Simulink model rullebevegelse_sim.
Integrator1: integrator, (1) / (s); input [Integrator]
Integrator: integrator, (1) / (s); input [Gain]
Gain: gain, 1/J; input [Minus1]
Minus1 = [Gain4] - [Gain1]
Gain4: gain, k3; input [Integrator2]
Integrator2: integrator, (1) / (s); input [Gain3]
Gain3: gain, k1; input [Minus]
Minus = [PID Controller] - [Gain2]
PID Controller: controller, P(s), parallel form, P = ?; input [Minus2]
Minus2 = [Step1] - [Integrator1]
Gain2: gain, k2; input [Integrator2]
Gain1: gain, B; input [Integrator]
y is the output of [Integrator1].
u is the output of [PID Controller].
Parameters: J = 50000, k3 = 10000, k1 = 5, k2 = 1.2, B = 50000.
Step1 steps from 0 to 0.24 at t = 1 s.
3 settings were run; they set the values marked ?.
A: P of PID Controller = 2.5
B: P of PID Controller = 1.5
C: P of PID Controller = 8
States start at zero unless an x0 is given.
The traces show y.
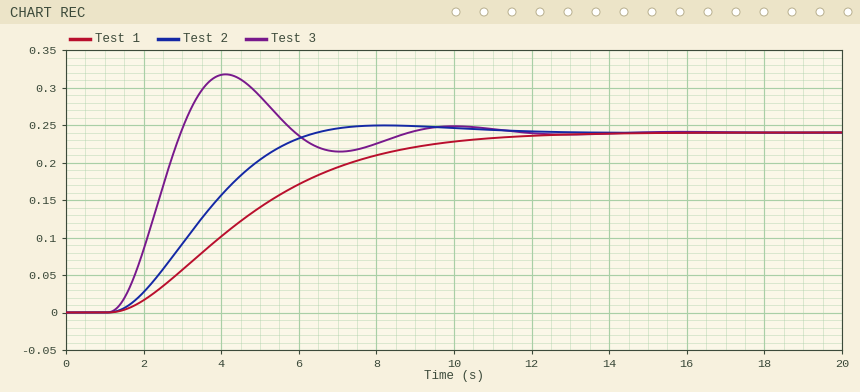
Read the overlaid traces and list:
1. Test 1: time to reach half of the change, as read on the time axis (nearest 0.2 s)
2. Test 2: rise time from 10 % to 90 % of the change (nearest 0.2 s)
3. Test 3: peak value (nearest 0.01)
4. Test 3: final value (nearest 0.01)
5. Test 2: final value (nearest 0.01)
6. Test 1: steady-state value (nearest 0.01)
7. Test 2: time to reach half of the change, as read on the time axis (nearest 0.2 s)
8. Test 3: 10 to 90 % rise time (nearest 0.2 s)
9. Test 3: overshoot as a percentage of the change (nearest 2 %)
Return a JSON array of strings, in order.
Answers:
["4.4 s", "3.4 s", "0.32", "0.24", "0.24", "0.24", "3.4 s", "1.2 s", "32 %"]
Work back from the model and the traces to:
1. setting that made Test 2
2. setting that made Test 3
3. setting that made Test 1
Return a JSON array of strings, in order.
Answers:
["A", "C", "B"]
